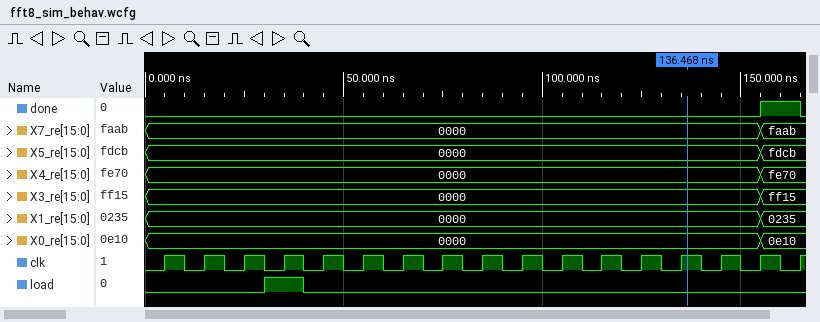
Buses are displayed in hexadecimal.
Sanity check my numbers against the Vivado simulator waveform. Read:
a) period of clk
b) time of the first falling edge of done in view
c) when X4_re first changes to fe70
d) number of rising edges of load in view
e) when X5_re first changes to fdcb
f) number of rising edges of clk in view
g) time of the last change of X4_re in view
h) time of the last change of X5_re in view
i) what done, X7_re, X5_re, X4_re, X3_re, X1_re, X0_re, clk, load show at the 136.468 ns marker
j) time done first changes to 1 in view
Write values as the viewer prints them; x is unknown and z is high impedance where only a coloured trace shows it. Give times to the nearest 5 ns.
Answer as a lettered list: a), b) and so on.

a) 10 ns
b) 165 ns
c) 155 ns
d) 1
e) 155 ns
f) 17
g) 155 ns
h) 155 ns
i) done=0, X7_re=0000, X5_re=0000, X4_re=0000, X3_re=0000, X1_re=0000, X0_re=0000, clk=1, load=0
j) 155 ns
